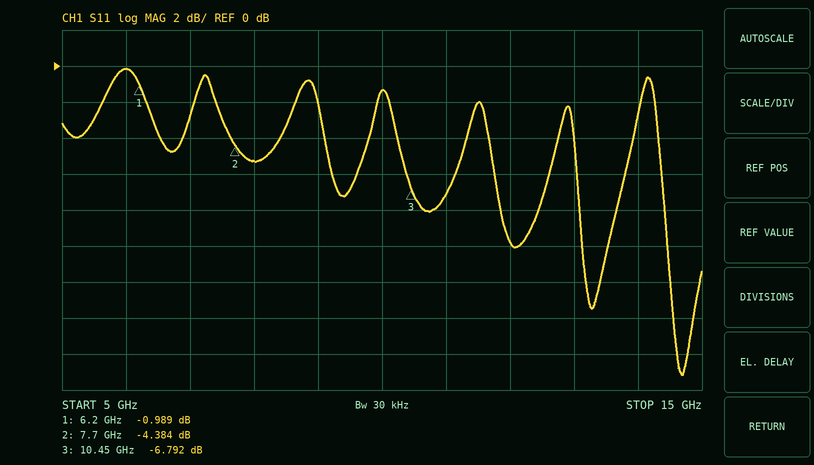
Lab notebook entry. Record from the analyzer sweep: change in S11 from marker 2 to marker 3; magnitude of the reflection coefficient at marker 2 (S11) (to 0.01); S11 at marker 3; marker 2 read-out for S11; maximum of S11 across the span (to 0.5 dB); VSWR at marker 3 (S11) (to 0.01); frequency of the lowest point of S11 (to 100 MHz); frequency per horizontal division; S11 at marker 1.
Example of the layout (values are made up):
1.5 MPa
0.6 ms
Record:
-2.408 dB
0.60
-6.792 dB
-4.384 dB
0.0 dB
2.69
14.7 GHz
1 GHz
-0.989 dB
